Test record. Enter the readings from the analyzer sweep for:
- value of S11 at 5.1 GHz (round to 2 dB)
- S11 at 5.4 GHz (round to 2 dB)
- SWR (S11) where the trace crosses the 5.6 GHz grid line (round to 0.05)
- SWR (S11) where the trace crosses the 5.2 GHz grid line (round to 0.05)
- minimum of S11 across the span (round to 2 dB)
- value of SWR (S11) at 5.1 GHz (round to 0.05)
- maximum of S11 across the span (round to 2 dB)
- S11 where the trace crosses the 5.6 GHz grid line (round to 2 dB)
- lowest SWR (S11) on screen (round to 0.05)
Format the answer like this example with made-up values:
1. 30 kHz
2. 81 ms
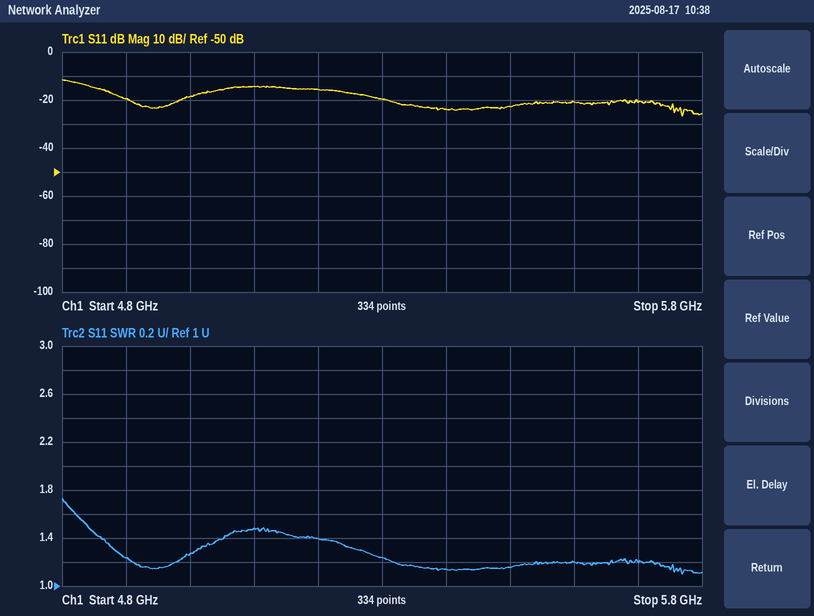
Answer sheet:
1. -14 dB
2. -24 dB
3. 1.20
4. 1.40
5. -26 dB
6. 1.50
7. -12 dB
8. -20 dB
9. 1.10
